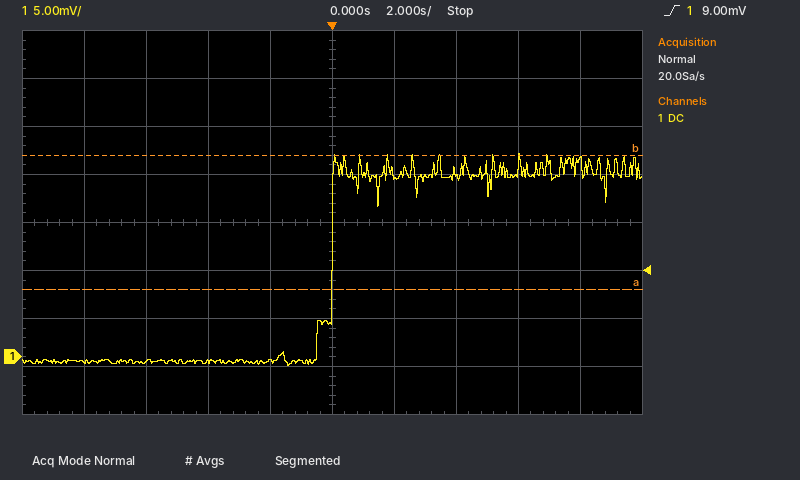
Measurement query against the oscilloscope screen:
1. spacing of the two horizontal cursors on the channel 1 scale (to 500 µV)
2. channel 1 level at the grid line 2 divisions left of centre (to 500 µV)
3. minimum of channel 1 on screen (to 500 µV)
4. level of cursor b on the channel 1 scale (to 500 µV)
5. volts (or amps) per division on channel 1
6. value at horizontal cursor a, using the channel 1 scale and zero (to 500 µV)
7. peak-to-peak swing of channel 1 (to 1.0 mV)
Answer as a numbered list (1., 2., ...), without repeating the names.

1. 14.0 mV
2. -500 µV
3. -1.0 mV
4. 21.0 mV
5. 5 mV
6. 7.0 mV
7. 22.0 mV
